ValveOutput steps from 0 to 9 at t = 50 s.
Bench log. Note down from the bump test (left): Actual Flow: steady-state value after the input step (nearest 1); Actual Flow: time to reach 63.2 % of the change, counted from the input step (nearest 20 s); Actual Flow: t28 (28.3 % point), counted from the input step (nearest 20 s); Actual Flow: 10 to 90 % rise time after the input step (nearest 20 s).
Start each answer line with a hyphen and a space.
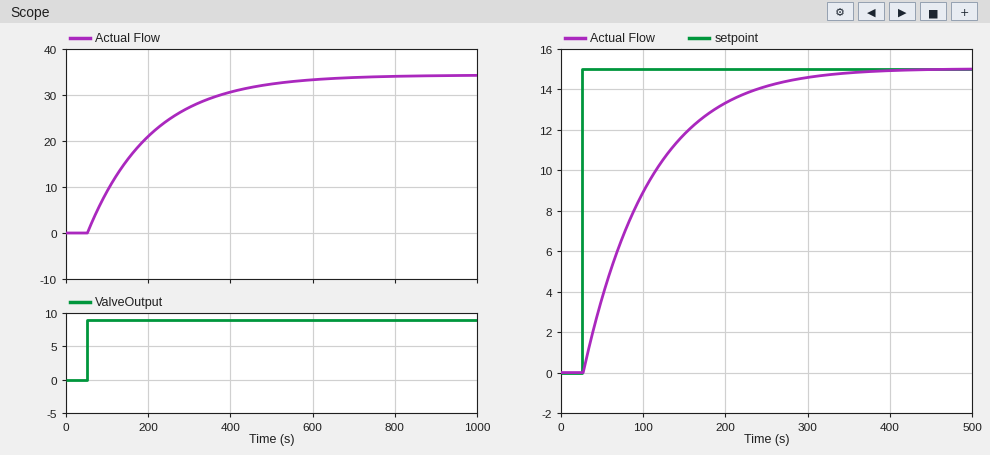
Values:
- 34
- 160 s
- 60 s
- 340 s
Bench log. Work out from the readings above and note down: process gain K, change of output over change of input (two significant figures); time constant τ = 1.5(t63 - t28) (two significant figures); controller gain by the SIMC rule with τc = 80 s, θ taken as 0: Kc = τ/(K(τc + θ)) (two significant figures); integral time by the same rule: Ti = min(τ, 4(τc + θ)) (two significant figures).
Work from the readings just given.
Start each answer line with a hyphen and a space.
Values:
- 3.8
- 150 s
- 0.49
- 150 s
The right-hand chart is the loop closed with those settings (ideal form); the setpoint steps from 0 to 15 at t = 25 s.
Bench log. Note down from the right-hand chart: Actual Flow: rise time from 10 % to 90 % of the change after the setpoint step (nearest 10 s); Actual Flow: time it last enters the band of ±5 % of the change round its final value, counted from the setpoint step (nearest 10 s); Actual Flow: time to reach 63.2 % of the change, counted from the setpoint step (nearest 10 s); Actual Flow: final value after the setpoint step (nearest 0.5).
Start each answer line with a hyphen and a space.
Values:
- 170 s
- 230 s
- 80 s
- 15.0
